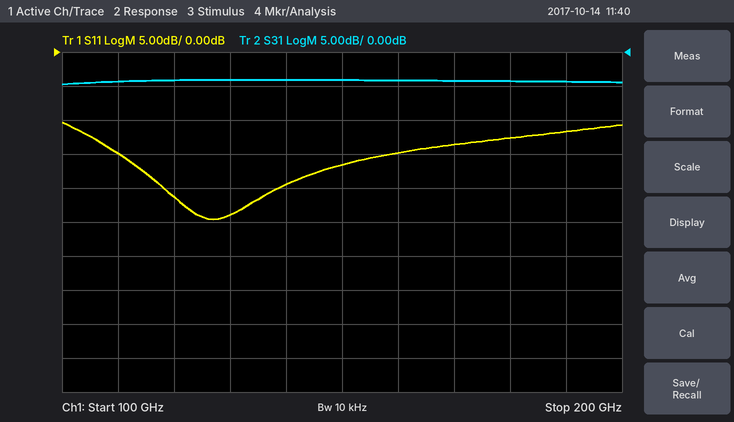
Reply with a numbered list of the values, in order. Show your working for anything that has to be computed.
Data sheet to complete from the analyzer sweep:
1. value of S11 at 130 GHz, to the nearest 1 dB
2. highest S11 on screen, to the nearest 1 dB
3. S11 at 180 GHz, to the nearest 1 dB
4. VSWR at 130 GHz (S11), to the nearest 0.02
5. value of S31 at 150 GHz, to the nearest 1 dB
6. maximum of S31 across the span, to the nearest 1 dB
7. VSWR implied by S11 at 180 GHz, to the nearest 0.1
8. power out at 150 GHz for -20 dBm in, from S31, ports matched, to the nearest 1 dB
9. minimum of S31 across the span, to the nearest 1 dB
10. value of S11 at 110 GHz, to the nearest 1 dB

1. -24 dB
2. -10 dB
3. -13 dB
4. |Γ| = 10^(-24/20) = 0.0631; VSWR = (1 + 0.0631)/(1 − 0.0631) ≈ 1.13, so 1.14 to the nearest 0.02
5. -4 dB
6. -4 dB
7. |Γ| = 10^(-13/20) = 0.2239; VSWR = (1 + 0.2239)/(1 − 0.2239) ≈ 1.6
8. -20 dBm + (-4 dB) = -24 dBm
9. -5 dB
10. -15 dB
